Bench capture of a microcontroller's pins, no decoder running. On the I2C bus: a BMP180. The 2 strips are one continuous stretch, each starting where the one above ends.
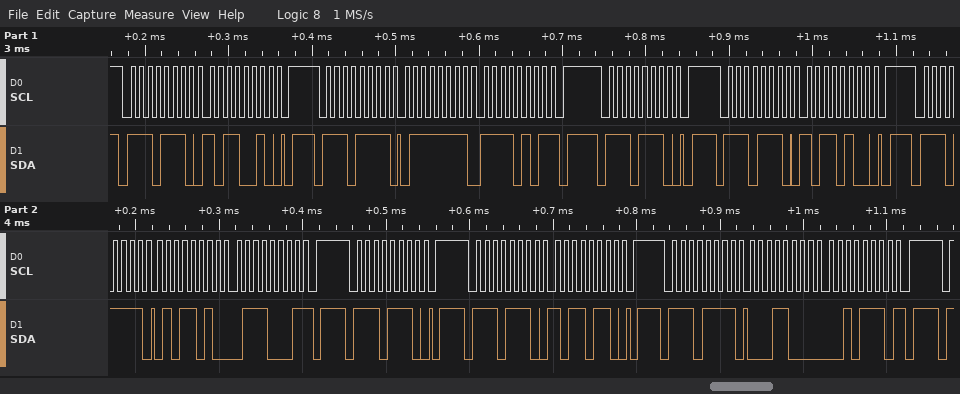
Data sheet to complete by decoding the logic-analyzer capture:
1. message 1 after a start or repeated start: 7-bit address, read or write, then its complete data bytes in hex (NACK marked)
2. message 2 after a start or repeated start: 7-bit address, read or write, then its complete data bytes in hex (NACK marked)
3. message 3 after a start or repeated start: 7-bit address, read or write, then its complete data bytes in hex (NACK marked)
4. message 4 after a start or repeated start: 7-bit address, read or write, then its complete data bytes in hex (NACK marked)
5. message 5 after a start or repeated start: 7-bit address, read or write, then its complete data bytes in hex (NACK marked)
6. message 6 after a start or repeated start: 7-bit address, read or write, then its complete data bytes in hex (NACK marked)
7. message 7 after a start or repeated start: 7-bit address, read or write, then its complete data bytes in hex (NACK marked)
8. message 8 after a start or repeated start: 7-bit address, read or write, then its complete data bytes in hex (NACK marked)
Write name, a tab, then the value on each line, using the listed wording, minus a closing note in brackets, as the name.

message 1 after a start or repeated start: 7-bit address, read or write, then its complete data bytes in hex	0x77 write: B2
message 2 after a start or repeated start: 7-bit address, read or write, then its complete data bytes in hex	0x77 read: 7F F5 NACK
message 3 after a start or repeated start: 7-bit address, read or write, then its complete data bytes in hex	0x77 write
message 4 after a start or repeated start: 7-bit address, read or write, then its complete data bytes in hex	0x77 write: B4
message 5 after a start or repeated start: 7-bit address, read or write, then its complete data bytes in hex	0x77 read: 5A 71 NACK
message 6 after a start or repeated start: 7-bit address, read or write, then its complete data bytes in hex	0x77 write
message 7 after a start or repeated start: 7-bit address, read or write, then its complete data bytes in hex	0x77 write: B6
message 8 after a start or repeated start: 7-bit address, read or write, then its complete data bytes in hex	0x77 read: 18 2E NACK
